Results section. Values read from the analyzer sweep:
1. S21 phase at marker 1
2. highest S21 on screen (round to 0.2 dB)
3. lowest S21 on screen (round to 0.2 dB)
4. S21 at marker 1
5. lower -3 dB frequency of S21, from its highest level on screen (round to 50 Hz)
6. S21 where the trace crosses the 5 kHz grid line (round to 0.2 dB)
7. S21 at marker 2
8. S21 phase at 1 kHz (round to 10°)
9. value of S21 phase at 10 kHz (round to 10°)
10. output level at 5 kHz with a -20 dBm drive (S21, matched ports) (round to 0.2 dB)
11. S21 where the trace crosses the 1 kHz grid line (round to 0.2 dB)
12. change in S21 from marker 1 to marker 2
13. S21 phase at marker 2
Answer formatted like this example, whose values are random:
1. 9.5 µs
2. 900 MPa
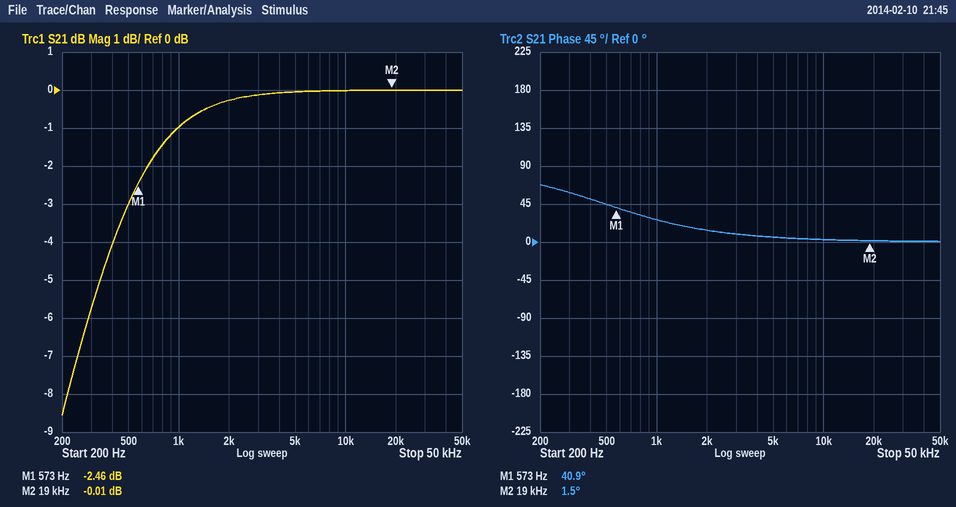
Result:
1. 40.9°
2. 0.0 dB
3. -8.6 dB
4. -2.46 dB
5. 500 Hz
6. 0.0 dB
7. -0.01 dB
8. 30°
9. 0°
10. -20.0 dBm
11. -1.0 dB
12. 2.45 dB
13. 1.5°
